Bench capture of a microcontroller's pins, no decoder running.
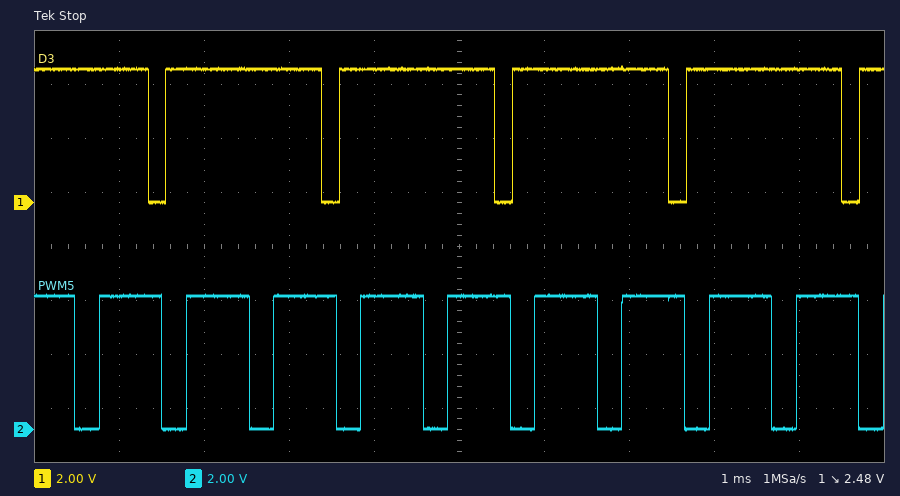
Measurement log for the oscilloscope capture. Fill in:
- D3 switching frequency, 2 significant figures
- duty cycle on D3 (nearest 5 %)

490 Hz
90 %
